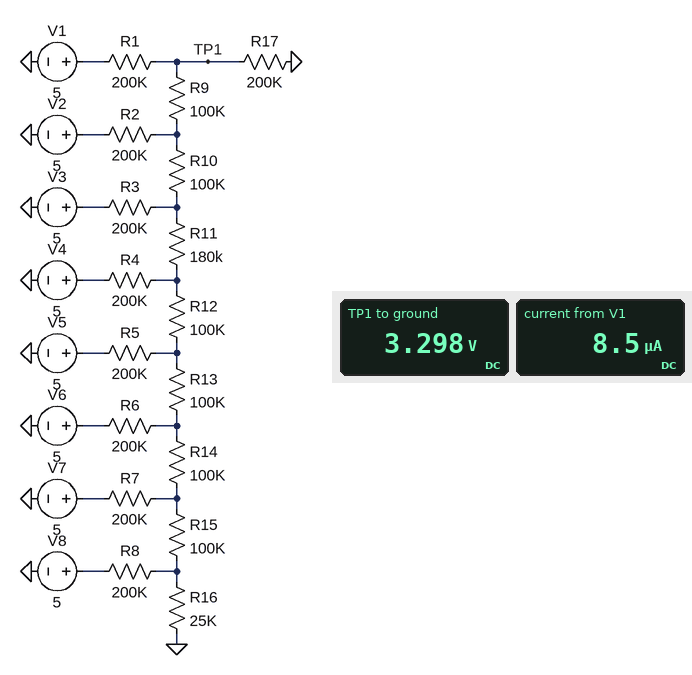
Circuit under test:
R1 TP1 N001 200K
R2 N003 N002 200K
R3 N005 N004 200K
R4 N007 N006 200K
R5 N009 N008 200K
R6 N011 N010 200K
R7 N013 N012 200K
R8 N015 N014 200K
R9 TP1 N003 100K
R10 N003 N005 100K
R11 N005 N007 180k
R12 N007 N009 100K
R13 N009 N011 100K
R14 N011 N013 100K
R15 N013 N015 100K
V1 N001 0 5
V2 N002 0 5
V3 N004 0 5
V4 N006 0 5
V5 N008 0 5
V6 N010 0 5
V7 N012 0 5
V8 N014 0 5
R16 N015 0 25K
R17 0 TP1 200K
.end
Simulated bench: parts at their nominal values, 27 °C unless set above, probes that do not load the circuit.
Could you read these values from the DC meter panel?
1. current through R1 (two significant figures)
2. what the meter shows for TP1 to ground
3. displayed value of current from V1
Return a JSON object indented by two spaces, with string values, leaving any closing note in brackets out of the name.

{
  "current through R1": "8.5 µA",
  "what the meter shows for TP1 to ground": "3.298 V",
  "displayed value of current from V1": "8.5 µA"
}
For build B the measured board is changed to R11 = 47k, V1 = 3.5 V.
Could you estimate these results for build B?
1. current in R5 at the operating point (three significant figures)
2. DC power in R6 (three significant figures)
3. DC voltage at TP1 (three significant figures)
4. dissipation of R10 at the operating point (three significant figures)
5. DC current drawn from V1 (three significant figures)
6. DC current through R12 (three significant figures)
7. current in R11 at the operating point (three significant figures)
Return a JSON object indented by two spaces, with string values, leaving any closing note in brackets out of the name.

{
  "current in R5 at the operating point": "3.25 µA",
  "DC power in R6": "5.75 µW",
  "DC voltage at TP1": "2.81 V",
  "dissipation of R10 at the operating point": "2.45 µW",
  "DC current drawn from V1": "3.45 µA",
  "DC current through R12": "981 nA",
  "current in R11 at the operating point": "1.78 µA"
}
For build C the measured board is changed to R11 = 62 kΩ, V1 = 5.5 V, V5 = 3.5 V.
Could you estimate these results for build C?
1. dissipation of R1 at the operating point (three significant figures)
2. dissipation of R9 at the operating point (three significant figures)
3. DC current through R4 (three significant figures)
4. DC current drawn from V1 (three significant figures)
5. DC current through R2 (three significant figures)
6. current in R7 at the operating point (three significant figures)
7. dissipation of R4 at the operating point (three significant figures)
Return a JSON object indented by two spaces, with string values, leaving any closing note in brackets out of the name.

{
  "dissipation of R1 at the operating point": "21.3 µW",
  "dissipation of R9 at the operating point": "4.70 µW",
  "DC current through R4": "3.38 µA",
  "DC current drawn from V1": "10.3 µA",
  "DC current through R2": "4.39 µA",
  "current in R7 at the operating point": "10.6 µA",
  "dissipation of R4 at the operating point": "2.28 µW"
}
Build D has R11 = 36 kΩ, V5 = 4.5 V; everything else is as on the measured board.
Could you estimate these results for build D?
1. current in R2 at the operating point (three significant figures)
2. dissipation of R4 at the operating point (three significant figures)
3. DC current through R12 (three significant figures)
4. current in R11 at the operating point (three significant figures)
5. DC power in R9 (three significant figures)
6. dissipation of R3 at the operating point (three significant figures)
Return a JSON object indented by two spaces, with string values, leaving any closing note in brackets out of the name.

{
  "current in R2 at the operating point": "4.55 µA",
  "dissipation of R4 at the operating point": "1.52 µW",
  "DC current through R12": "2.22 µA",
  "current in R11 at the operating point": "539 nA",
  "DC power in R9": "6.32 µW",
  "dissipation of R3 at the operating point": "1.63 µW"
}
